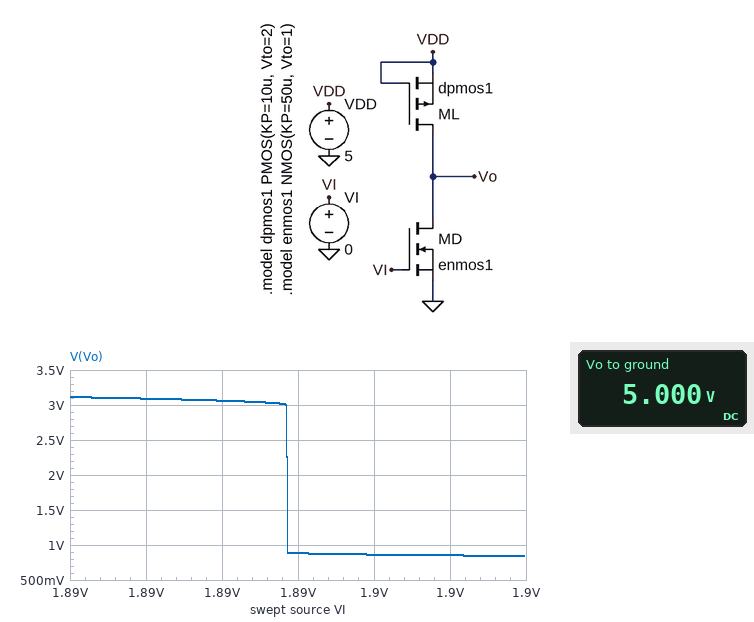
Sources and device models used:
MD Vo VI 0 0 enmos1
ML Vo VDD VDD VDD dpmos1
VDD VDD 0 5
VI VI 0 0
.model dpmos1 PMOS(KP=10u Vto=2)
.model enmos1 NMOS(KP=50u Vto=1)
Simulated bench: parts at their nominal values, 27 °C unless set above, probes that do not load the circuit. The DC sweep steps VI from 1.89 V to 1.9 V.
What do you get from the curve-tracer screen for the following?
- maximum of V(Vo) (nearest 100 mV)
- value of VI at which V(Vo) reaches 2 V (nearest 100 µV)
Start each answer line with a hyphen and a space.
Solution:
- 3.1 V
- 1.8944 V
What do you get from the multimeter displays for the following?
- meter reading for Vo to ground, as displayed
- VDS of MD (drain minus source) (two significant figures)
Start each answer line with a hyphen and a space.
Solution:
- 5.000 V
- 5.0 V
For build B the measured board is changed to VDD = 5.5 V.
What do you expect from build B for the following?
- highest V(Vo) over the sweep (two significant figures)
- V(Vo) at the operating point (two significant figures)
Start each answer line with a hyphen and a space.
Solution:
- 3.6 V
- 5.5 V
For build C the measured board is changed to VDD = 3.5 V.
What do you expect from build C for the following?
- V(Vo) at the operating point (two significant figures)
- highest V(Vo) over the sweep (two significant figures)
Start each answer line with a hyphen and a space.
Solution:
- 3.5 V
- 1.6 V
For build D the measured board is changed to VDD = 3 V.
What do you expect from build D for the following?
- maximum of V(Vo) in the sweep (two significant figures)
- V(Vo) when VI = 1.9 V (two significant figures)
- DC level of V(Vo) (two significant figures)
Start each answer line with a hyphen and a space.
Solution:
- 1.1 V
- 850 mV
- 3.0 V
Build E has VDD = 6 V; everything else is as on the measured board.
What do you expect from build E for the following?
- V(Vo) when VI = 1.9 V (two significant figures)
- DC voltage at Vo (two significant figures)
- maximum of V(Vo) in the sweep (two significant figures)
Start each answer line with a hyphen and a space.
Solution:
- 850 mV
- 6.0 V
- 4.1 V
